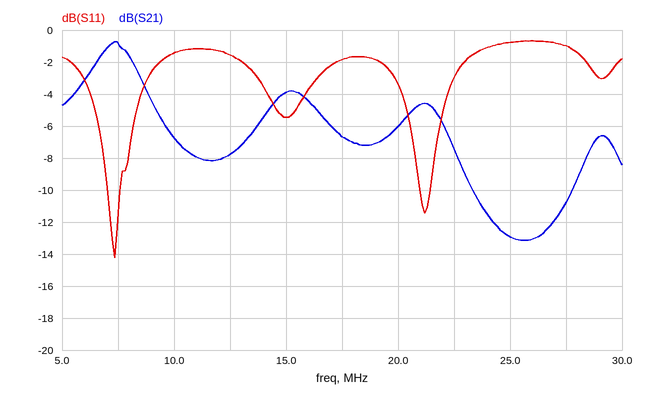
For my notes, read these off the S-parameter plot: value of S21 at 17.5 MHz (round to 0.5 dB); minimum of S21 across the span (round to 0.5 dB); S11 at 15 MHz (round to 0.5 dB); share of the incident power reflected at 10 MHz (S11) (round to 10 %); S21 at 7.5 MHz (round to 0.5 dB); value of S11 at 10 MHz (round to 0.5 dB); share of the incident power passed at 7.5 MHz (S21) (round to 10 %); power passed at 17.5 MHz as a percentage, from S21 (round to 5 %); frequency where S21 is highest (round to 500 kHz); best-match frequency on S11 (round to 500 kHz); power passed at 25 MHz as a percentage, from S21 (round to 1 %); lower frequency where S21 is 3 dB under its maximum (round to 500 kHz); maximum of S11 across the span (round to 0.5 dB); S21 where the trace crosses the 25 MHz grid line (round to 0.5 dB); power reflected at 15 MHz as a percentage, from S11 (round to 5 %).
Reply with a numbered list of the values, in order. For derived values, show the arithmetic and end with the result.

1. -6.5 dB
2. -13.0 dB
3. -5.5 dB
4. 10^(-1.5/10) ≈ 70.8 %, so 70 % to the nearest 10 %
5. -1.0 dB
6. -1.5 dB
7. 10^(-1/10) ≈ 79.4 %, so 80 % to the nearest 10 %
8. 10^(-6.5/10) ≈ 22.4 %, so 20 % to the nearest 5 %
9. 7.5 MHz
10. 7.5 MHz
11. 10^(-13/10) ≈ 5 %
12. 5.5 MHz
13. -0.5 dB
14. -13.0 dB
15. 10^(-5.5/10) ≈ 28.2 %, so 30 % to the nearest 5 %
